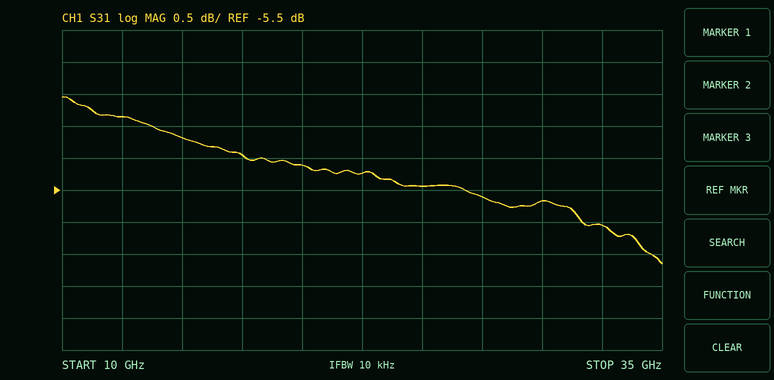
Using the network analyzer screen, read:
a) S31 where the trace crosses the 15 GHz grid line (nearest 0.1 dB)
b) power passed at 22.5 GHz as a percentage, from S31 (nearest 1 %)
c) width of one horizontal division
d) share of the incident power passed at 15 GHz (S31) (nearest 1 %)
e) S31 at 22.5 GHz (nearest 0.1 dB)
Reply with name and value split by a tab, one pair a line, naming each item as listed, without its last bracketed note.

S31 where the trace crosses the 15 GHz grid line	-4.7 dB
power passed at 22.5 GHz as a percentage, from S31	30 %
width of one horizontal division	2.5 GHz
share of the incident power passed at 15 GHz (S31)	34 %
S31 at 22.5 GHz	-5.2 dB
